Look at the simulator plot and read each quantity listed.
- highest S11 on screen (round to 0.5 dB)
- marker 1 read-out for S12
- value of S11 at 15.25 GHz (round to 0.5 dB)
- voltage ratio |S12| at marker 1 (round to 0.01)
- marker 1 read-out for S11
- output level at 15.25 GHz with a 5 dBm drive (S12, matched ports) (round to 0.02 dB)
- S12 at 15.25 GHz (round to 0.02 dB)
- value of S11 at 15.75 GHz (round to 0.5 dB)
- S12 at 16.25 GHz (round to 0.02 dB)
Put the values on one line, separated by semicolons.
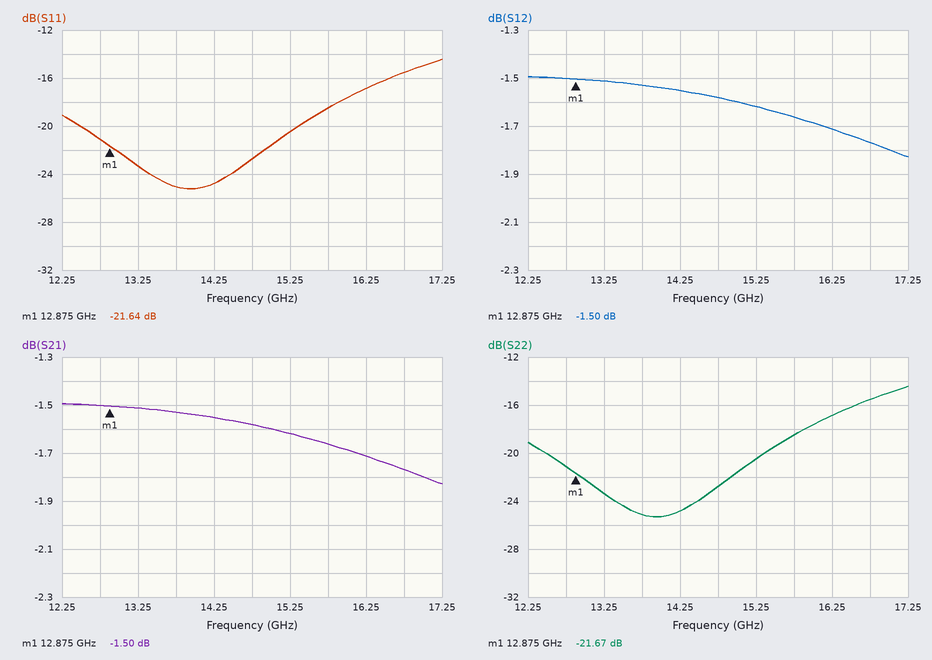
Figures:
-14.5 dB; -1.50 dB; -20.5 dB; 0.84; -21.64 dB; 3.38 dBm; -1.62 dB; -18.5 dB; -1.72 dB
